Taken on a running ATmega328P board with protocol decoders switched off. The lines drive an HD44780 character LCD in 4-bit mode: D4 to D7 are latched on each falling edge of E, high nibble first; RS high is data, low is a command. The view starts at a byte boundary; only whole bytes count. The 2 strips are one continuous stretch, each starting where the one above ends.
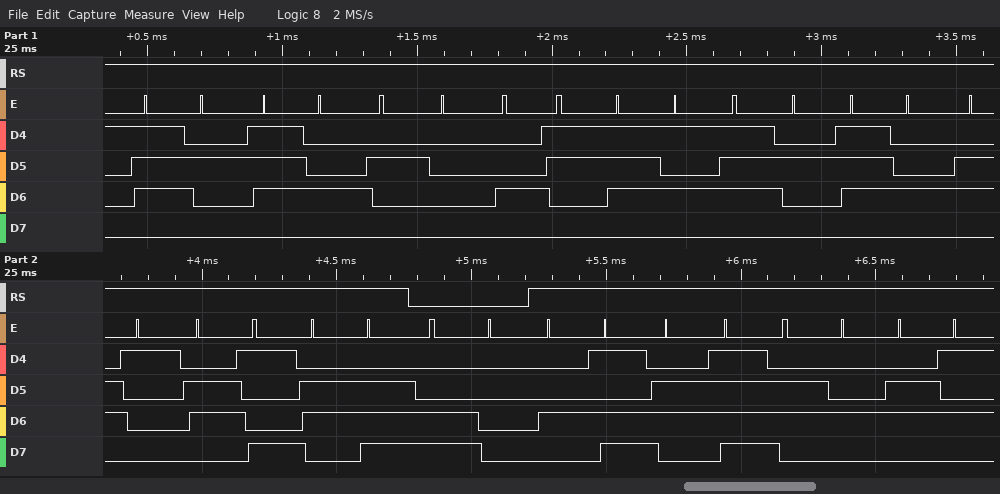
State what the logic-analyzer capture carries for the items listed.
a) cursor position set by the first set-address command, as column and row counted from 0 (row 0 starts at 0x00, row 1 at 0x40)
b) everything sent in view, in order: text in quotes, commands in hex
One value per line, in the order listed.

column 0, row 1
"rt Curtain" 0xC0 "Mode"
